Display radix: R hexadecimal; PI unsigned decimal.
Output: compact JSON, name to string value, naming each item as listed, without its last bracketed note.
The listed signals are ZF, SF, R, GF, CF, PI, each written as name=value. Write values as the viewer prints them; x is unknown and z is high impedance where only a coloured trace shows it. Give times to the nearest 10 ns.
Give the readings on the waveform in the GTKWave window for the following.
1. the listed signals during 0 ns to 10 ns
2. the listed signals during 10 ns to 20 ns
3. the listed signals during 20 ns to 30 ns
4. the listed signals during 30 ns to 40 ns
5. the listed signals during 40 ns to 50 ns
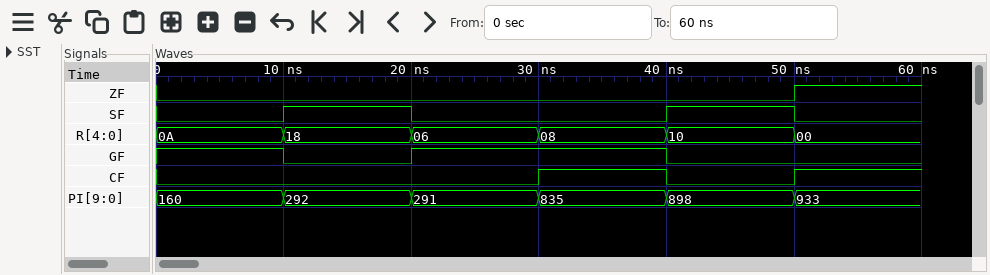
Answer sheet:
{"the listed signals during 0 ns to 10 ns": "ZF=0, SF=0, R=0A, GF=1, CF=0, PI=160", "the listed signals during 10 ns to 20 ns": "ZF=0, SF=1, R=18, GF=0, CF=0, PI=292", "the listed signals during 20 ns to 30 ns": "ZF=0, SF=0, R=06, GF=1, CF=0, PI=291", "the listed signals during 30 ns to 40 ns": "ZF=0, SF=0, R=08, GF=1, CF=1, PI=835", "the listed signals during 40 ns to 50 ns": "ZF=0, SF=1, R=10, GF=0, CF=0, PI=898"}
